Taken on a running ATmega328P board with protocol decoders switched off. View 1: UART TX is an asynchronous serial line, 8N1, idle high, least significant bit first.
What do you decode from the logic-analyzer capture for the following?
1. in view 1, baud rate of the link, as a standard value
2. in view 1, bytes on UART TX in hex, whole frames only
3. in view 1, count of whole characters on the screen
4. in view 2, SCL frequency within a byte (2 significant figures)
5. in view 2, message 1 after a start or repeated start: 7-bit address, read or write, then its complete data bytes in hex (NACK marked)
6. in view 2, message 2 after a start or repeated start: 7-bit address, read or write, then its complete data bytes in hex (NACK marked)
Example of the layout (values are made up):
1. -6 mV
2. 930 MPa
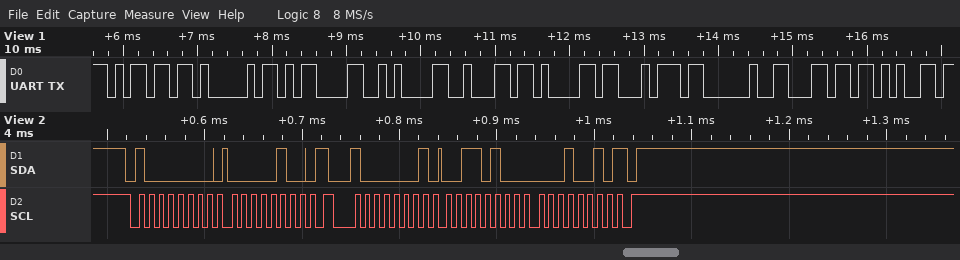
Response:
1. 9600 baud
2. 0x6D 0x41 0x0D 0x0A 0x62 0x61 0x74 0x20 0x6C 0x65
3. 10
4. 100 kHz
5. 0x40 write: 04
6. 0x40 read: 34 12 NACK
